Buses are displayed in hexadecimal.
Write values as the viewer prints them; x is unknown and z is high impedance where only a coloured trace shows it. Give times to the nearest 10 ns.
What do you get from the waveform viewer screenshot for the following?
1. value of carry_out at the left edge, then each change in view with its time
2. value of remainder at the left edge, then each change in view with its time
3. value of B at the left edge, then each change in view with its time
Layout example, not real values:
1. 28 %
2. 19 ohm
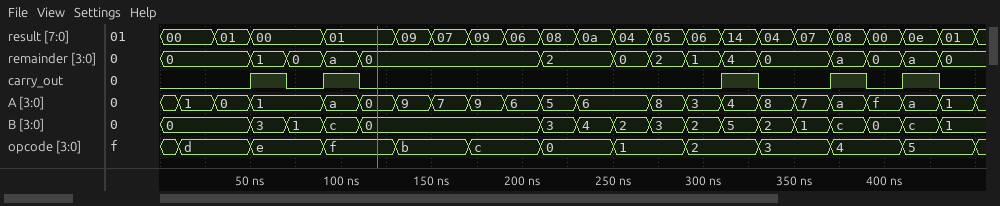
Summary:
1. 0, 1 at 50 ns, 0 at 70 ns, 1 at 90 ns, 0 at 110 ns, 1 at 310 ns, 0 at 330 ns, 1 at 370 ns, 0 at 390 ns, 1 at 410 ns, 0 at 430 ns
2. 0, 1 at 50 ns, 0 at 70 ns, a at 90 ns, 0 at 110 ns, 2 at 210 ns, 0 at 250 ns, 2 at 270 ns, 1 at 290 ns, 4 at 310 ns, 0 at 330 ns, a at 370 ns, 0 at 390 ns, a at 410 ns, 0 at 430 ns
3. 0, 3 at 50 ns, 1 at 70 ns, c at 90 ns, 0 at 110 ns, 3 at 210 ns, 4 at 230 ns, 2 at 250 ns, 3 at 270 ns, 2 at 290 ns, 5 at 310 ns, 2 at 330 ns, 1 at 350 ns, c at 370 ns, 0 at 390 ns, c at 410 ns, 1 at 430 ns
